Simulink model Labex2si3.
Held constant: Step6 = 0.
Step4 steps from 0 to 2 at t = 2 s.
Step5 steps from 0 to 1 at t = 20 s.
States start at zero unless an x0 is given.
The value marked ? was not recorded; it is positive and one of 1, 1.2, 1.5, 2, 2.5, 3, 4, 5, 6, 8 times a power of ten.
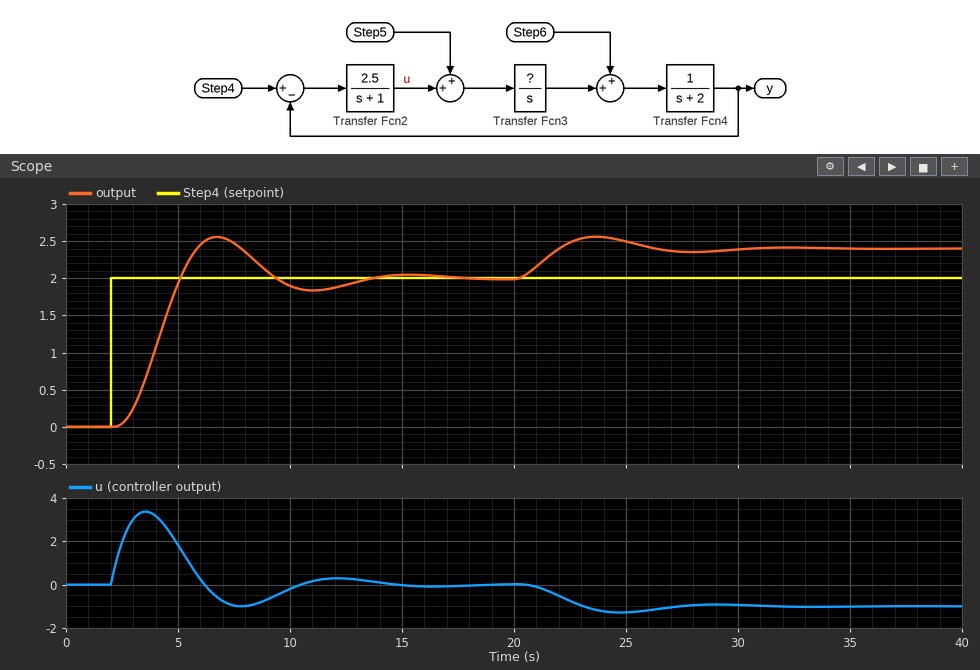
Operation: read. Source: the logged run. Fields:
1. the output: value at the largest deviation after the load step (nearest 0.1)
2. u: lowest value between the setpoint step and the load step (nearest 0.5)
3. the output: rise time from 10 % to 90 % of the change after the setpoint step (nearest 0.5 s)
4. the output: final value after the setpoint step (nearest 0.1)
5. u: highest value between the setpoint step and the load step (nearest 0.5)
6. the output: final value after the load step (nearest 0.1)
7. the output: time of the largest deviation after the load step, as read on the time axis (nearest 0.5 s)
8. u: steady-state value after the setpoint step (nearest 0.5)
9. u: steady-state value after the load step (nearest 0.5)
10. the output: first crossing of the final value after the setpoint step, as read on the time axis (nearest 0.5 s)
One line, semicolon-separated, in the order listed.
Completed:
2.6; -1.0; 2.0 s; 2.0; 3.5; 2.4; 23.5 s; 0.0; -1.0; 5.0 s
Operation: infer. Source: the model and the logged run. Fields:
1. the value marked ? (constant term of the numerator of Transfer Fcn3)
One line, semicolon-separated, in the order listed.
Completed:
0.6
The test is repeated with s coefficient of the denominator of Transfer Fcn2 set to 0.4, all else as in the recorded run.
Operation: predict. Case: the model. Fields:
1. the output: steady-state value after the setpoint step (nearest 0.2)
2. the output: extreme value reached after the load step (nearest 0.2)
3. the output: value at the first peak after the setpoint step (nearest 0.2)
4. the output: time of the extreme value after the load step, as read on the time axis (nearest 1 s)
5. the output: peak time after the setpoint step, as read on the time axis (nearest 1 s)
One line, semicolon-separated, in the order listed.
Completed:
2.0; 2.4; 2.2; 23 s; 6 s
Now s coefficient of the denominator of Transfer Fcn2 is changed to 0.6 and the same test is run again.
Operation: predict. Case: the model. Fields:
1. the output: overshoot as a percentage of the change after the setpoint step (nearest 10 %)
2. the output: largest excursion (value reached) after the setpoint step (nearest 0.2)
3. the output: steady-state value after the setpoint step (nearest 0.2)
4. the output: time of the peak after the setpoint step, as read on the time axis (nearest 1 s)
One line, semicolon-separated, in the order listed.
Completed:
20 %; 2.4; 2.0; 6 s
